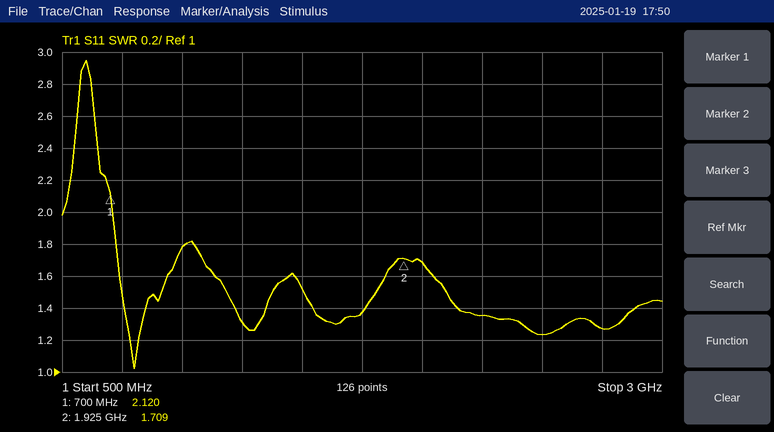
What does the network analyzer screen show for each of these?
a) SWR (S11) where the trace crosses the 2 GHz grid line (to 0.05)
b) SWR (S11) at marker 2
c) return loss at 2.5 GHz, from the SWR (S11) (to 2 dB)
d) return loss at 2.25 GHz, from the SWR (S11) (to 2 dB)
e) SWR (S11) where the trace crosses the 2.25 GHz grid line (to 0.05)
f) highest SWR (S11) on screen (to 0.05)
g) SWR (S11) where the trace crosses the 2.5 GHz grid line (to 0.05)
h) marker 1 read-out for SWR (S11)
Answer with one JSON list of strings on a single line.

["1.70", "1.709", "20 dB", "16 dB", "1.35", "2.95", "1.25", "2.120"]
